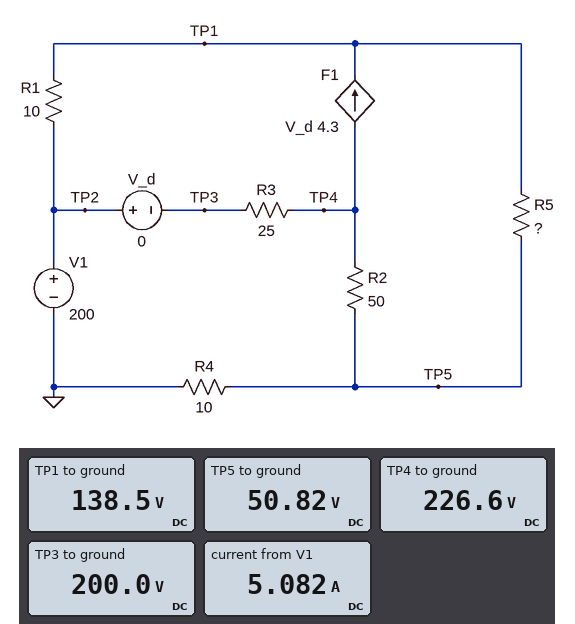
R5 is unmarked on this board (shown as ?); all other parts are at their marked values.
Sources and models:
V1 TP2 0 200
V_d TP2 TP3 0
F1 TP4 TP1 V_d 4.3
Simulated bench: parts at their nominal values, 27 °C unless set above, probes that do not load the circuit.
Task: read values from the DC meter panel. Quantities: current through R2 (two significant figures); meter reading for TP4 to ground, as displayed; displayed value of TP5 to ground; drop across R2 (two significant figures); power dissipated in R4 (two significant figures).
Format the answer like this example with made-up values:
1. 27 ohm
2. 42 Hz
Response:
1. 3.5 A
2. 226.6 V
3. 50.82 V
4. 180 V
5. 260 W
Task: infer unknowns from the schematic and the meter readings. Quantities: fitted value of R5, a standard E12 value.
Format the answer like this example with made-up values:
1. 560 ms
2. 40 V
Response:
1. 56 Ω
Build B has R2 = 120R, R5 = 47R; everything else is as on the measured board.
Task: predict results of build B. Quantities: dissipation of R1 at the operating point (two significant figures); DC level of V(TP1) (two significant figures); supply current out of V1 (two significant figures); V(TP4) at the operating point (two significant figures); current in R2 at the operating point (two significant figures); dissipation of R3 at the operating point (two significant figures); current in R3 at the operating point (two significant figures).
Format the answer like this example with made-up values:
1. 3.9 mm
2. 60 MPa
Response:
1. 190 W
2. 160 V
3. 3.9 A
4. 210 V
5. 1.4 A
6. 4.7 W
7. 430 mA
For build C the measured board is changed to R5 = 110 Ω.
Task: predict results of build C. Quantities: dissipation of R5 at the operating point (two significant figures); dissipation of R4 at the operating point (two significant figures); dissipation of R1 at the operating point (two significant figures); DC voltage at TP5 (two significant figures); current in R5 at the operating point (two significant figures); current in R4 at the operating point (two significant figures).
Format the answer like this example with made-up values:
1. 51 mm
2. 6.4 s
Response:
1. 88 W
2. 210 W
3. 320 W
4. 45 V
5. 890 mA
6. 4.5 A
